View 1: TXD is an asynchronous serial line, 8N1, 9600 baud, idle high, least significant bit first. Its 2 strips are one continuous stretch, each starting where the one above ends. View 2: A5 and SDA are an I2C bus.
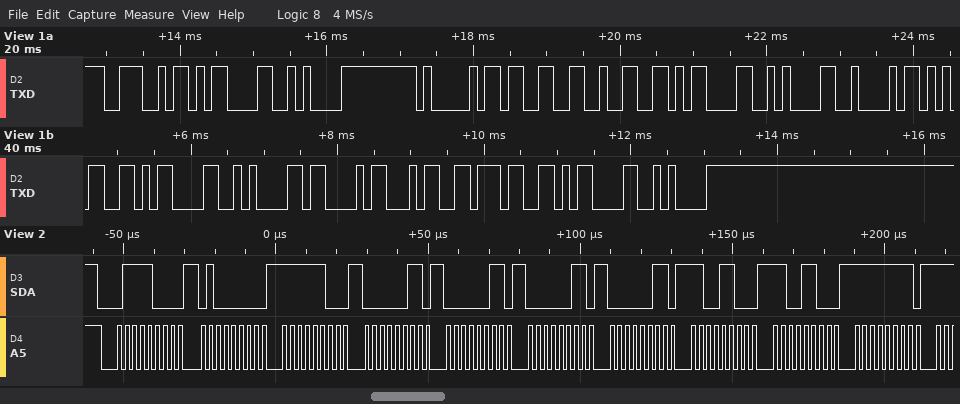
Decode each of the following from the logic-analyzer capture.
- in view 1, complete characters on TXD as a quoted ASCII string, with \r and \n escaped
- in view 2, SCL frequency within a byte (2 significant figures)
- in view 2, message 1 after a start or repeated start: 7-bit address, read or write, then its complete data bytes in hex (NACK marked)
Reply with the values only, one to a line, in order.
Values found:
"N\r\nA32\r\nB5\r\nC47\r\n"
400 kHz
0x3C write: 40 FC 03 03 03 03 CC CC FF
